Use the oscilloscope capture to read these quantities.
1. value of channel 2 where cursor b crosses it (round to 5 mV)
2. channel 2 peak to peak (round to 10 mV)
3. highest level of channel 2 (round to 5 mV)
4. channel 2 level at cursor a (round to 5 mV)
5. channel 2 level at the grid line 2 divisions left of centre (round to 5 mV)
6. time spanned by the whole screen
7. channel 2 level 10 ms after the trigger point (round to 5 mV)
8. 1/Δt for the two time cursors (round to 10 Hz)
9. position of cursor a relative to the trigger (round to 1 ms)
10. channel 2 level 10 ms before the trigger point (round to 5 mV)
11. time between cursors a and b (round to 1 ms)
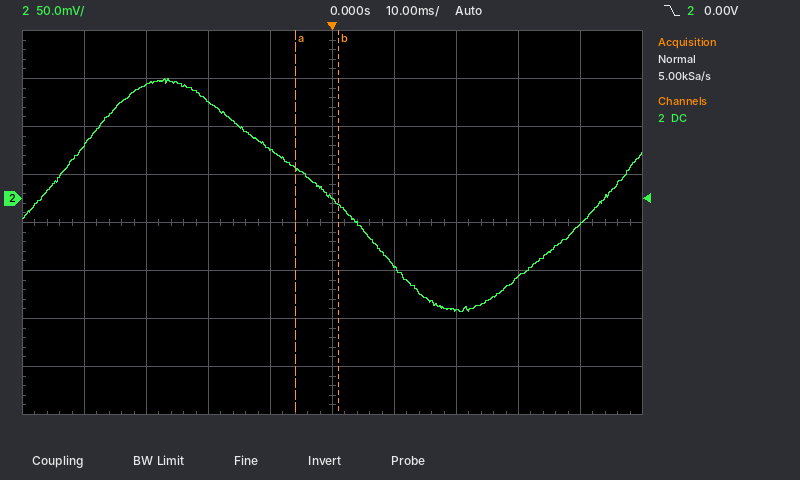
-5 mV
240 mV
125 mV
30 mV
100 mV
100 ms
-70 mV
140 Hz
-6 ms
50 mV
7 ms
